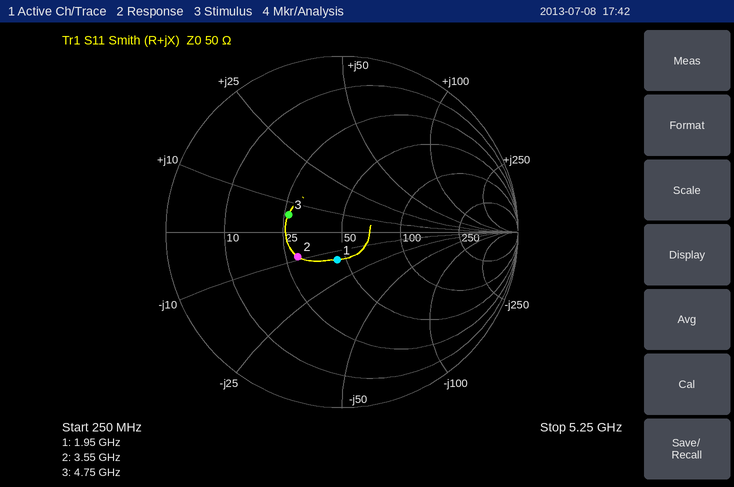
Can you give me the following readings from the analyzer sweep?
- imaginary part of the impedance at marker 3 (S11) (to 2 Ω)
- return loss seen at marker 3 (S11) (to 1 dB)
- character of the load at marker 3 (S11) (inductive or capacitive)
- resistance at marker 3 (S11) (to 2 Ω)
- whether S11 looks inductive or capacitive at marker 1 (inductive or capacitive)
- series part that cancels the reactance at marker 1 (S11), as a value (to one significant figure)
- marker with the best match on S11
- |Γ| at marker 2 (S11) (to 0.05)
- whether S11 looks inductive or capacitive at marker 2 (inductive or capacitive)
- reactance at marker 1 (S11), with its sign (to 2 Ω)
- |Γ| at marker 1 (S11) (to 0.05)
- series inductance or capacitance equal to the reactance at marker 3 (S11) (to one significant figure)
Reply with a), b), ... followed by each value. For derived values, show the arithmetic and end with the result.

a) +6 Ω
b) 10 dB
c) inductive
d) 26 Ω
e) capacitive
f) L = 14 Ω/(2π × 1.95 GHz) ≈ 1 nH
g) marker 1
h) 0.30
i) capacitive
j) -14 Ω
k) 0.15
l) L = 6 Ω/(2π × 4.75 GHz) ≈ 201 pH, so 200 pH to one significant figure
